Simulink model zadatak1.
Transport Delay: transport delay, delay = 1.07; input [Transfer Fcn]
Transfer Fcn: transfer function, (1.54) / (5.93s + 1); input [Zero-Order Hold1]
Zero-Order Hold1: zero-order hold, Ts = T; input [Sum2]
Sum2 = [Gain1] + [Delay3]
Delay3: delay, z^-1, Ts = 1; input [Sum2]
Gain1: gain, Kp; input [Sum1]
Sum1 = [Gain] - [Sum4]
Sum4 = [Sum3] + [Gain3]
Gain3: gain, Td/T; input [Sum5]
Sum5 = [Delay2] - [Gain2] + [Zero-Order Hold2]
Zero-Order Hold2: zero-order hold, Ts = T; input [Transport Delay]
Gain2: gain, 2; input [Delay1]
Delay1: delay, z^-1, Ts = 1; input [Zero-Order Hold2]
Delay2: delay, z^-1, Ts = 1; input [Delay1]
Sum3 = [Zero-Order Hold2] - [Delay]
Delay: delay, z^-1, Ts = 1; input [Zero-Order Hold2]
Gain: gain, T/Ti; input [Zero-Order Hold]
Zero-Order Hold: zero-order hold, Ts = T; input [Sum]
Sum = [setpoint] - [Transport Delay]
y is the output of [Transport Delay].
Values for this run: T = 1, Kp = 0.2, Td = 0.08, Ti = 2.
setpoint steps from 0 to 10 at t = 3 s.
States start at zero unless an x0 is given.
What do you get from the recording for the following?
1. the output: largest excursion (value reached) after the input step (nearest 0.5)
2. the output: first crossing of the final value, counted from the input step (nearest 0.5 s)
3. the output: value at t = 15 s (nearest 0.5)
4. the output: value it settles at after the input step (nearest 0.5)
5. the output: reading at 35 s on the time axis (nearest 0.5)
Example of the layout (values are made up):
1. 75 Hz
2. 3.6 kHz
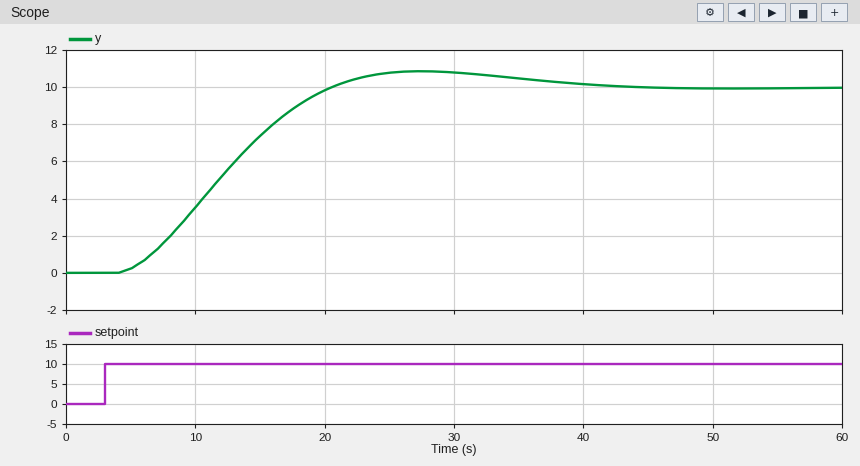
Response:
1. 11.0
2. 17.5 s
3. 7.5
4. 10.0
5. 10.5
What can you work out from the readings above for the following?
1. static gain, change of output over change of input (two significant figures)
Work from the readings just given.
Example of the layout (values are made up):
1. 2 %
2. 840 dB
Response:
1. 1.0
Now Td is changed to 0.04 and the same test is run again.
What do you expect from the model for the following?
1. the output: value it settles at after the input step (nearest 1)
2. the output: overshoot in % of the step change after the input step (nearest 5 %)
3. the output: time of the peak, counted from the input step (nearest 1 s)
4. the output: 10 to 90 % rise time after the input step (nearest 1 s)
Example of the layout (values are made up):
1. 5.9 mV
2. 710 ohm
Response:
1. 10
2. 10 %
3. 24 s
4. 11 s
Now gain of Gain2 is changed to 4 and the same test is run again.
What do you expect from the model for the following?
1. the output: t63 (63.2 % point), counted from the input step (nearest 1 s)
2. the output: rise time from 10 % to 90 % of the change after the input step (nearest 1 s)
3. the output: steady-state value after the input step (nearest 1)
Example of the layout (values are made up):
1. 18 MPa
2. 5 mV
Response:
1. 14 s
2. 18 s
3. 15
